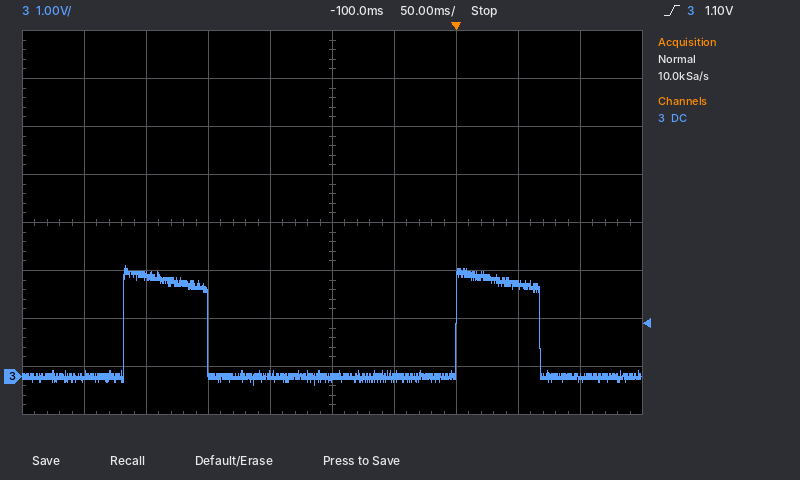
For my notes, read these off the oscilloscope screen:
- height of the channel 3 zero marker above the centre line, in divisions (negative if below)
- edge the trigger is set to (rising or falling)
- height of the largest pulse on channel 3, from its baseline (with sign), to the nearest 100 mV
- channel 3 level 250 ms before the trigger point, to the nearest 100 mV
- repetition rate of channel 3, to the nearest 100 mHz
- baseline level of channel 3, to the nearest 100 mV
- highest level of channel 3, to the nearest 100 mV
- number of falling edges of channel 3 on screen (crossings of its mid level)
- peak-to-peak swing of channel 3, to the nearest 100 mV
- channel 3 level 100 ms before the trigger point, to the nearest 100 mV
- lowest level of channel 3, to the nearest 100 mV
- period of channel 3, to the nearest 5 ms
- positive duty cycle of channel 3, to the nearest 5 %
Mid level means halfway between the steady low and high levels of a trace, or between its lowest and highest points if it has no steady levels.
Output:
-3.2 div
rising
+2.3 V
2.1 V
3.7 Hz
0.0 V
2.3 V
2
2.5 V
0.0 V
-200 mV
270 ms
25 %
